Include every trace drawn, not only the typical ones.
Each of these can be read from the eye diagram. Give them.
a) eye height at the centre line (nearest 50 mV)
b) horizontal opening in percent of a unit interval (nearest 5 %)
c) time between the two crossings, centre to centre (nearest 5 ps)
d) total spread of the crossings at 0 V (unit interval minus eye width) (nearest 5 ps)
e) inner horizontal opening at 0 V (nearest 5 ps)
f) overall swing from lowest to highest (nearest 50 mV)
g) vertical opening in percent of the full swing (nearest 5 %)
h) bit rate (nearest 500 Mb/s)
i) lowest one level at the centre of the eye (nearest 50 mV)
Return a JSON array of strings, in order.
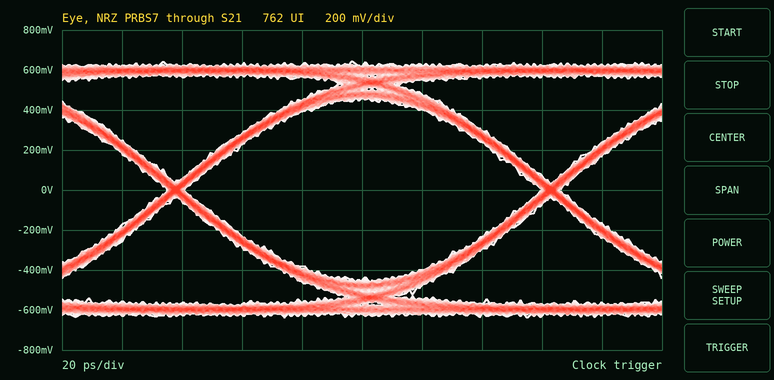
["900 mV", "95 %", "125 ps", "5 ps", "120 ps", "1.30 V", "70 %", "8.0 Gb/s", "450 mV"]
